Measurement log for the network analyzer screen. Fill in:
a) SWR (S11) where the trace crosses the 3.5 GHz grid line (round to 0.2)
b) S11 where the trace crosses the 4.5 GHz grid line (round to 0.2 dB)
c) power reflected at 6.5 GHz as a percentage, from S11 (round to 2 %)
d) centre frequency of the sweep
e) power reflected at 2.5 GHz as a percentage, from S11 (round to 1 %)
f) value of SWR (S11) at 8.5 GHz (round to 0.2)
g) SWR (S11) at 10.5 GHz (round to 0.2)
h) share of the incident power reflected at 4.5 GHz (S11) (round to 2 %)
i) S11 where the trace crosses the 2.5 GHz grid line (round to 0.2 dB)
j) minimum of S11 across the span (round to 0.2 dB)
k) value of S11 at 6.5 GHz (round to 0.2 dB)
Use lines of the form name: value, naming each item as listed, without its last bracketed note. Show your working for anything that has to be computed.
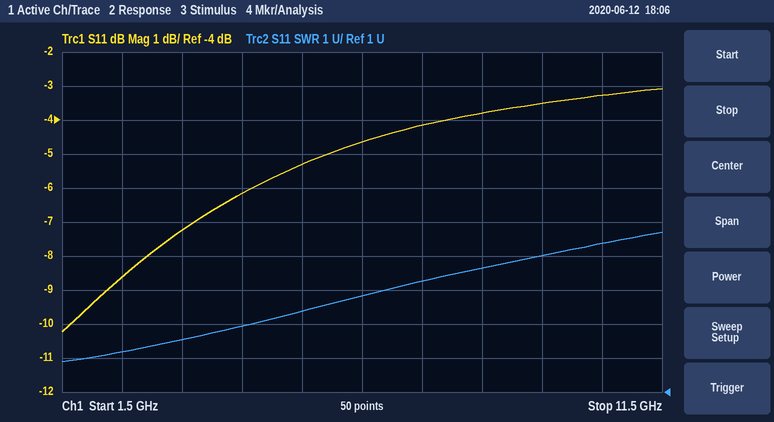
SWR (S11) where the trace crosses the 3.5 GHz grid line: 2.6
S11 where the trace crosses the 4.5 GHz grid line: -6.2 dB
power reflected at 6.5 GHz as a percentage, from S11: 10^(-4.6/10) ≈ 34.7 %, so 34 % to the nearest 2 %
centre frequency of the sweep: 6.5 GHz
power reflected at 2.5 GHz as a percentage, from S11: 10^(-8.6/10) ≈ 14 %
value of SWR (S11) at 8.5 GHz: 4.6
SWR (S11) at 10.5 GHz: 5.4
share of the incident power reflected at 4.5 GHz (S11): 10^(-6.2/10) ≈ 24 %
S11 where the trace crosses the 2.5 GHz grid line: -8.6 dB
minimum of S11 across the span: -10.2 dB
value of S11 at 6.5 GHz: -4.6 dB
